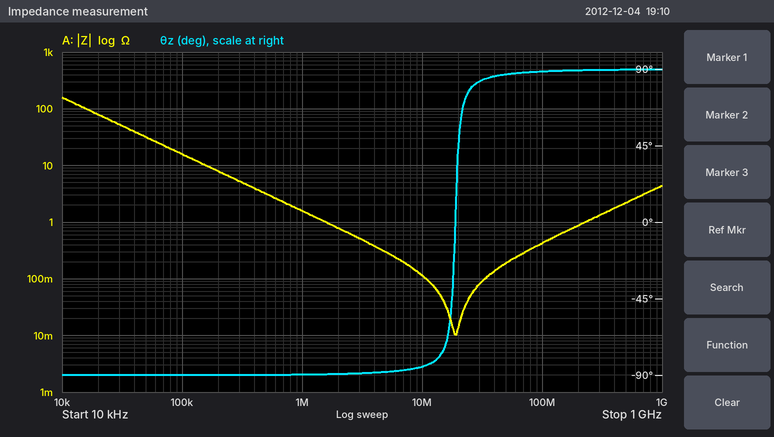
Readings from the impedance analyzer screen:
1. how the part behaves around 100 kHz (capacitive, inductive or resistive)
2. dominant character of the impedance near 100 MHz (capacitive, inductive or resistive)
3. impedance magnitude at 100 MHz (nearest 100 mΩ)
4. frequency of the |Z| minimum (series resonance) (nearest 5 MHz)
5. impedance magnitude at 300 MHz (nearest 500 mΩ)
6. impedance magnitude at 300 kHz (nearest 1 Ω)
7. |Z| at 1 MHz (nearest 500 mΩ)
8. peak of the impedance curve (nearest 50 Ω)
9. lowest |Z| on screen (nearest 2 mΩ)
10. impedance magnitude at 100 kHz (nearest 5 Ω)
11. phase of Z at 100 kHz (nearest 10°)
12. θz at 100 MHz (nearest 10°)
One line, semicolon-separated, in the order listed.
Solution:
capacitive; inductive; 400 mΩ; 20 MHz; 1.5 Ω; 5 Ω; 1.5 Ω; 150 Ω; 10 mΩ; 15 Ω; -90°; 90°
